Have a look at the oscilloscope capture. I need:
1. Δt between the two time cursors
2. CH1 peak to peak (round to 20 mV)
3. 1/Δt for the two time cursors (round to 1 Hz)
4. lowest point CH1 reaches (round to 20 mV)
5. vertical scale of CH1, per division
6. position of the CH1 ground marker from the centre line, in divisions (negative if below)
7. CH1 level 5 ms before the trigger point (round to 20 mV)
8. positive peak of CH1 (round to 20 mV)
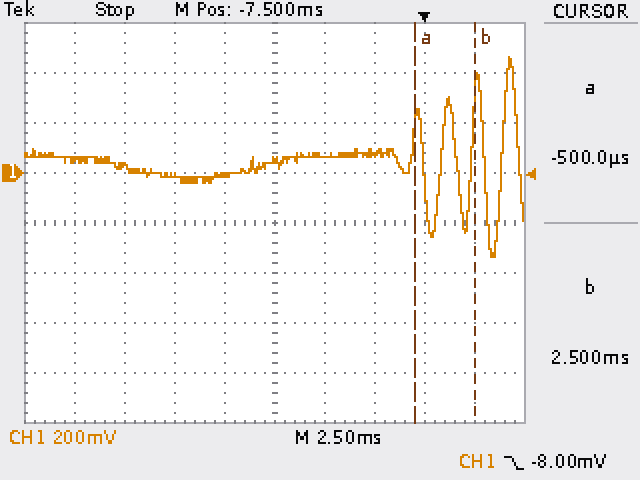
3.00 ms
800 mV
333 Hz
-340 mV
200 mV
+1.0 div
60 mV
460 mV
